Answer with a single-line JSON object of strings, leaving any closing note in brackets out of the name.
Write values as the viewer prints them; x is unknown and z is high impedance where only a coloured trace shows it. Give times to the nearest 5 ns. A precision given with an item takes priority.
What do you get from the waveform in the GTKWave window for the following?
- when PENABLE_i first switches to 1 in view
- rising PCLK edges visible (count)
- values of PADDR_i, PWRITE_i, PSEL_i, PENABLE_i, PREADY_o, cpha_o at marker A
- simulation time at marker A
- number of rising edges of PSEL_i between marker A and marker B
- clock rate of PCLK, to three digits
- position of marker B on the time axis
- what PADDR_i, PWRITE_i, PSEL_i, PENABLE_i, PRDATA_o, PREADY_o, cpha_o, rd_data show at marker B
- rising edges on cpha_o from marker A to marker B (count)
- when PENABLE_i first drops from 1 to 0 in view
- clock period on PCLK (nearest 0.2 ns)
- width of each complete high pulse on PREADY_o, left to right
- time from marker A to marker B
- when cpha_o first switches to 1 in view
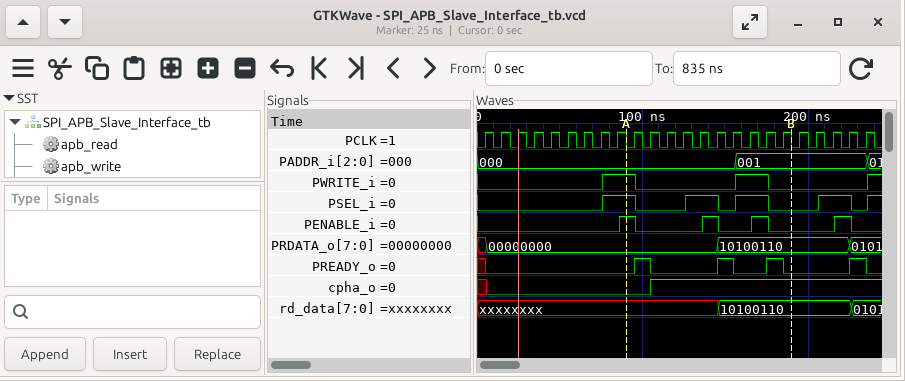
{"when PENABLE_i first switches to 1 in view": "85 ns", "rising PCLK edges visible": "24", "values of PADDR_i, PWRITE_i, PSEL_i, PENABLE_i, PREADY_o, cpha_o at marker A": "PADDR_i=000, PWRITE_i=1, PSEL_i=1, PENABLE_i=1, PREADY_o=0, cpha_o=0", "simulation time at marker A": "90 ns", "number of rising edges of PSEL_i between marker A and marker B": "2", "clock rate of PCLK, to three digits": "100 MHz", "position of marker B on the time axis": "190 ns", "what PADDR_i, PWRITE_i, PSEL_i, PENABLE_i, PRDATA_o, PREADY_o, cpha_o, rd_data show at marker B": "PADDR_i=001, PWRITE_i=0, PSEL_i=0, PENABLE_i=0, PRDATA_o=10100110, PREADY_o=0, cpha_o=1, rd_data=10100110", "rising edges on cpha_o from marker A to marker B": "1", "when PENABLE_i first drops from 1 to 0 in view": "95 ns", "clock period on PCLK": "10 ns", "width of each complete high pulse on PREADY_o, left to right": "10 ns, 10 ns, 10 ns, 10 ns", "time from marker A to marker B": "100 ns", "when cpha_o first switches to 1 in view": "105 ns"}
